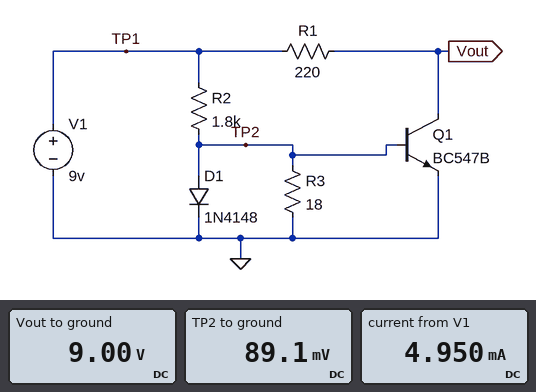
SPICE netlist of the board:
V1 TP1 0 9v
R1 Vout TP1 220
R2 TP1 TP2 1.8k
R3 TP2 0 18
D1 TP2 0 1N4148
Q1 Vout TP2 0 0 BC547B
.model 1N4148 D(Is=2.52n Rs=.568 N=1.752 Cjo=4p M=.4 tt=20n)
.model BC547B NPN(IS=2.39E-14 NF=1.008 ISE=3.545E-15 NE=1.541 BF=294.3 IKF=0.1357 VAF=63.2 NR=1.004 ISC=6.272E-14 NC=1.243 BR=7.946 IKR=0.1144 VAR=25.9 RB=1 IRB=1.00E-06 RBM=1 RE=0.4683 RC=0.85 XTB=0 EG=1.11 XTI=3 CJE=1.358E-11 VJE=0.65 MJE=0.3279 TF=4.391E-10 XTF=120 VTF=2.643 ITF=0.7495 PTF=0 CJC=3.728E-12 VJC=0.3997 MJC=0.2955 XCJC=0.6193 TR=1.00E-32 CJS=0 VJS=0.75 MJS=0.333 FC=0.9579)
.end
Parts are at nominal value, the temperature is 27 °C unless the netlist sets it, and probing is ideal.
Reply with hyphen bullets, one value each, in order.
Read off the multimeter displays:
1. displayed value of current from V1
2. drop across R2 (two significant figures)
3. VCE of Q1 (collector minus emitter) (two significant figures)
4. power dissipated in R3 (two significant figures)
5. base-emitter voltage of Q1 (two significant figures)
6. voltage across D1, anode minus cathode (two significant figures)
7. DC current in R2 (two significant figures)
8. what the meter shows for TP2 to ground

- 4.950 mA
- 8.9 V
- 9.0 V
- 440 µW
- 89 mV
- 89 mV
- 5.0 mA
- 89.1 mV
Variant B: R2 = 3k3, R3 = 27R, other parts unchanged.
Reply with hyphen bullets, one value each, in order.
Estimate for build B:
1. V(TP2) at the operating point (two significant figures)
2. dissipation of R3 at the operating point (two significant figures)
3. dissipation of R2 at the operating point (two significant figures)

- 73 mV
- 200 µW
- 24 mW
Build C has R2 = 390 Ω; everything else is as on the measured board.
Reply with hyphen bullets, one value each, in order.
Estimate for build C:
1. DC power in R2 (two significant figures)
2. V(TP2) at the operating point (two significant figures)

- 190 mW
- 400 mV
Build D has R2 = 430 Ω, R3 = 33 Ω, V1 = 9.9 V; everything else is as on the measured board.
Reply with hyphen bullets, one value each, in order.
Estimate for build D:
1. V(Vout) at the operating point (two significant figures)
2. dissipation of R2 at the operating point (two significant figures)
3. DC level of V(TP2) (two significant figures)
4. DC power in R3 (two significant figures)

- 9.7 V
- 200 mW
- 630 mV
- 12 mW
